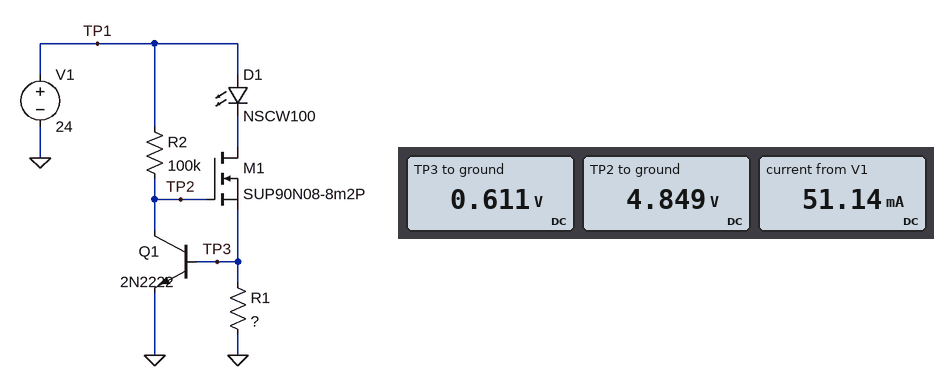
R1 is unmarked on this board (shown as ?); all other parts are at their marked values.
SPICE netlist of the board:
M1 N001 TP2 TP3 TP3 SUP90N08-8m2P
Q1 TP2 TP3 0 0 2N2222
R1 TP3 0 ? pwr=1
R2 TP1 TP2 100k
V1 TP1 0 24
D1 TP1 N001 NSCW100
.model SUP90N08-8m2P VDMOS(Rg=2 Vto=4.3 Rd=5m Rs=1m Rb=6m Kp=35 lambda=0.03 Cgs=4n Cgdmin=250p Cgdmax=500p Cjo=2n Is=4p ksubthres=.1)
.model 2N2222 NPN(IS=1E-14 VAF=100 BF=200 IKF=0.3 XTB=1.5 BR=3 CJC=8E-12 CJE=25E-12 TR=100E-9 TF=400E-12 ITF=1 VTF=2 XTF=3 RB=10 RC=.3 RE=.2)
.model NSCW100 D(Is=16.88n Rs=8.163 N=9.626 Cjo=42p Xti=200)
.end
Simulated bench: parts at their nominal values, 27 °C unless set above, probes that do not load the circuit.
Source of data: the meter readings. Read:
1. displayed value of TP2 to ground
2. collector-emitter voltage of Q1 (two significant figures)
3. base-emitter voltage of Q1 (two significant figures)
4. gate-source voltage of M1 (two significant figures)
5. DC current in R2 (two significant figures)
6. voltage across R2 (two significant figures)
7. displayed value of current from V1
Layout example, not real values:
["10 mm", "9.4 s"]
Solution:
["4.849 V", "4.8 V", "610 mV", "4.2 V", "190 µA", "19 V", "51.14 mA"]
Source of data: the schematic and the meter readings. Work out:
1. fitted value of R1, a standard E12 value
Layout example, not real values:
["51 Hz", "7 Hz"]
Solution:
["12 Ω"]
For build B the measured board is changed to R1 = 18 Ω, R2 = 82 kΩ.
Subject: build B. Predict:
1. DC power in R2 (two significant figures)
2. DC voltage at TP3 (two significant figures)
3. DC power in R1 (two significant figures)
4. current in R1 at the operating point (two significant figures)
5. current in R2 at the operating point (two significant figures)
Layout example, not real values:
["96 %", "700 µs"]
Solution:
["4.5 mW", "620 mV", "21 mW", "34 mA", "230 µA"]
